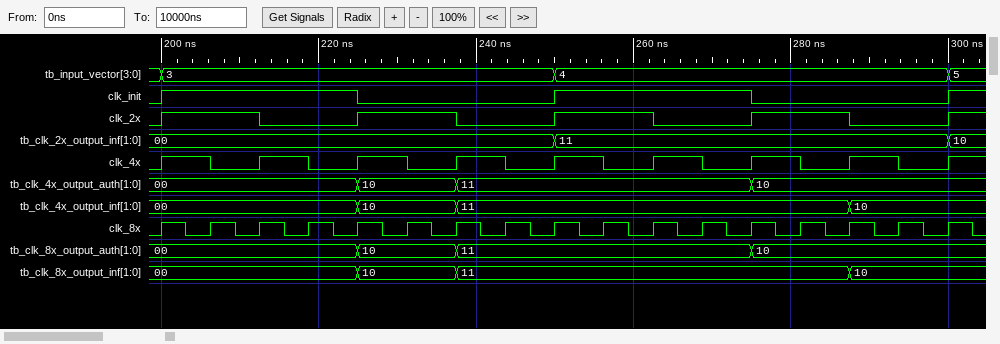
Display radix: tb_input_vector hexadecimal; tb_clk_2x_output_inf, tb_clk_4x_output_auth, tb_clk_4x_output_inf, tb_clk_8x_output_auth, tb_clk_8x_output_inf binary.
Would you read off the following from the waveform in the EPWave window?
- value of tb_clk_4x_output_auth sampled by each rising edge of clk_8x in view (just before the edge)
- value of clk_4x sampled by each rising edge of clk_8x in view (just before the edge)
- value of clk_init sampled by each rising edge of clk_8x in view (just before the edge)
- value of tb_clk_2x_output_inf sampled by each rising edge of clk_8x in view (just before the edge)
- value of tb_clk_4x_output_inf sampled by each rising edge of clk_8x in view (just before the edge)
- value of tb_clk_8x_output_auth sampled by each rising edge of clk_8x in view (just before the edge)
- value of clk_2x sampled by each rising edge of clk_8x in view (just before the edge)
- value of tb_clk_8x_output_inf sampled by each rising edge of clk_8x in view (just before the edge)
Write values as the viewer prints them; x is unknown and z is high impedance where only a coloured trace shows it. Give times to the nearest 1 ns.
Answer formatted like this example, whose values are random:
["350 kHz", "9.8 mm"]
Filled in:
["00, 00, 00, 00, 00, 10, 10, 11, 11, 11, 11, 11, 11, 10, 10, 10, 10", "0 1 0 1 0 1 0 1 0 1 0 1 0 1 0 1 0", "0 1 1 1 1 0 0 0 0 1 1 1 1 0 0 0 0", "00, 00, 00, 00, 00, 00, 00, 00, 00, 11, 11, 11, 11, 11, 11, 11, 11", "00, 00, 00, 00, 00, 10, 10, 11, 11, 11, 11, 11, 11, 11, 11, 10, 10", "00, 00, 00, 00, 00, 10, 10, 11, 11, 11, 11, 11, 11, 10, 10, 10, 10", "0 1 1 0 0 1 1 0 0 1 1 0 0 1 1 0 0", "00, 00, 00, 00, 00, 10, 10, 11, 11, 11, 11, 11, 11, 11, 11, 10, 10"]
